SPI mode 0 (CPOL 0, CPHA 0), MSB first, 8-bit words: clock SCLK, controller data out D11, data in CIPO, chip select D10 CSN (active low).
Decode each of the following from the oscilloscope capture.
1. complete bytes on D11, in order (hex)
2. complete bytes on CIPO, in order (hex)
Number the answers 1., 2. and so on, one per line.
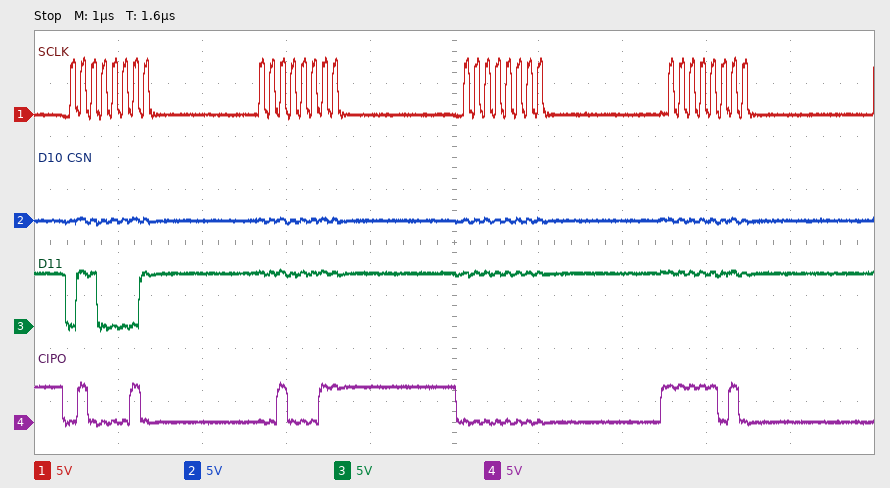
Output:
1. 61 FF FF FF
2. 42 23 00 FA
